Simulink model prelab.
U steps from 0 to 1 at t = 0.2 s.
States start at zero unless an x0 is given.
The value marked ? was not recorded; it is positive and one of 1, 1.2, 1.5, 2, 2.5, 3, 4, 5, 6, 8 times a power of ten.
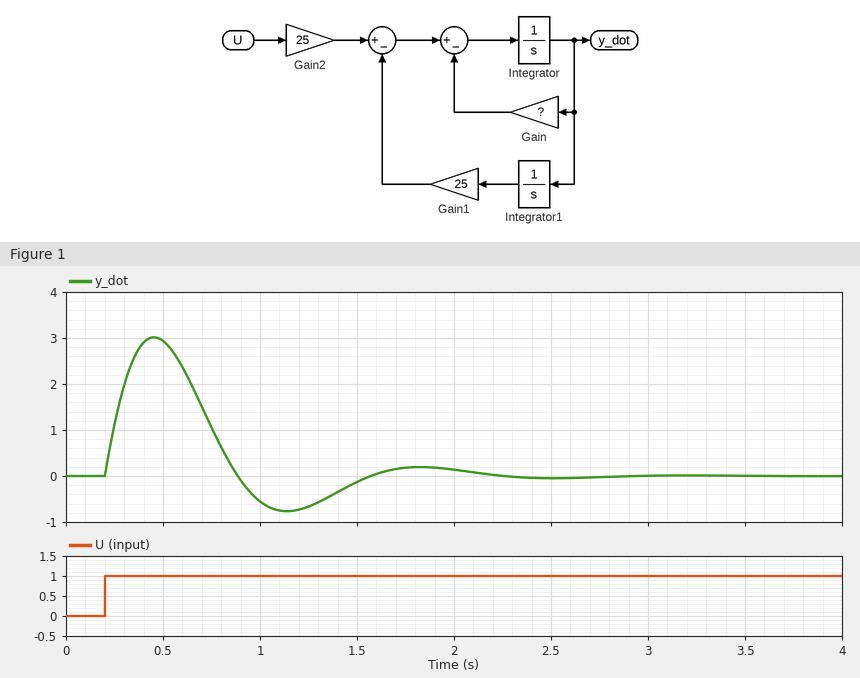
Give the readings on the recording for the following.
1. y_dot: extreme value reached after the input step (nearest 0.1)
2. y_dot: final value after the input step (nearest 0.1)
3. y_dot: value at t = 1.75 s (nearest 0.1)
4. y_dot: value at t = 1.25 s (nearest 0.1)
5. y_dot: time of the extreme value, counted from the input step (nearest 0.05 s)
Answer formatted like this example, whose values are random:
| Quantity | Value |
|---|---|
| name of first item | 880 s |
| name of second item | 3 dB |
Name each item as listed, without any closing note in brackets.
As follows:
| Quantity | Value |
|---|---|
| y_dot: extreme value reached after the input step | 3.0 |
| y_dot: final value after the input step | 0.0 |
| y_dot: value at t = 1.75 s | 0.2 |
| y_dot: value at t = 1.25 s | -0.7 |
| y_dot: time of the extreme value, counted from the input step | 0.25 s |
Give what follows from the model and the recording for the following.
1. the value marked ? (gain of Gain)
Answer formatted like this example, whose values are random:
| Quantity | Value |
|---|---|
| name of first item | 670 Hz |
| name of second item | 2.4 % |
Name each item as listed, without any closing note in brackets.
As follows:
| Quantity | Value |
|---|---|
| the value marked ? | 4 |
